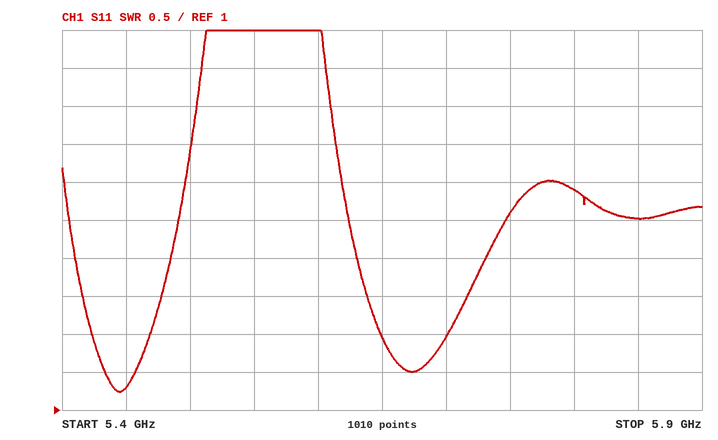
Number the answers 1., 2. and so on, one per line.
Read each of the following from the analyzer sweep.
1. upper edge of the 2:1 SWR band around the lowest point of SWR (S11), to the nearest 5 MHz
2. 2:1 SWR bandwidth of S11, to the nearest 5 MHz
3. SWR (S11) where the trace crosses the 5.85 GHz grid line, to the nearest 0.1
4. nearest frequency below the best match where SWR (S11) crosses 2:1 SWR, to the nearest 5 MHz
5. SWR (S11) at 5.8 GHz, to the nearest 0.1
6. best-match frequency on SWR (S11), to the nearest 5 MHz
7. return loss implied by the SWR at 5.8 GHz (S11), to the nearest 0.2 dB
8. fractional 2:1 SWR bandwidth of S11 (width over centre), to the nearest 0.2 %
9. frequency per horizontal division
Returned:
1. 5.470 GHz
2. 45 MHz
3. 3.5
4. 5.425 GHz
5. 3.9
6. 5.445 GHz
7. 4.6 dB
8. 0.8 %
9. 50 MHz
